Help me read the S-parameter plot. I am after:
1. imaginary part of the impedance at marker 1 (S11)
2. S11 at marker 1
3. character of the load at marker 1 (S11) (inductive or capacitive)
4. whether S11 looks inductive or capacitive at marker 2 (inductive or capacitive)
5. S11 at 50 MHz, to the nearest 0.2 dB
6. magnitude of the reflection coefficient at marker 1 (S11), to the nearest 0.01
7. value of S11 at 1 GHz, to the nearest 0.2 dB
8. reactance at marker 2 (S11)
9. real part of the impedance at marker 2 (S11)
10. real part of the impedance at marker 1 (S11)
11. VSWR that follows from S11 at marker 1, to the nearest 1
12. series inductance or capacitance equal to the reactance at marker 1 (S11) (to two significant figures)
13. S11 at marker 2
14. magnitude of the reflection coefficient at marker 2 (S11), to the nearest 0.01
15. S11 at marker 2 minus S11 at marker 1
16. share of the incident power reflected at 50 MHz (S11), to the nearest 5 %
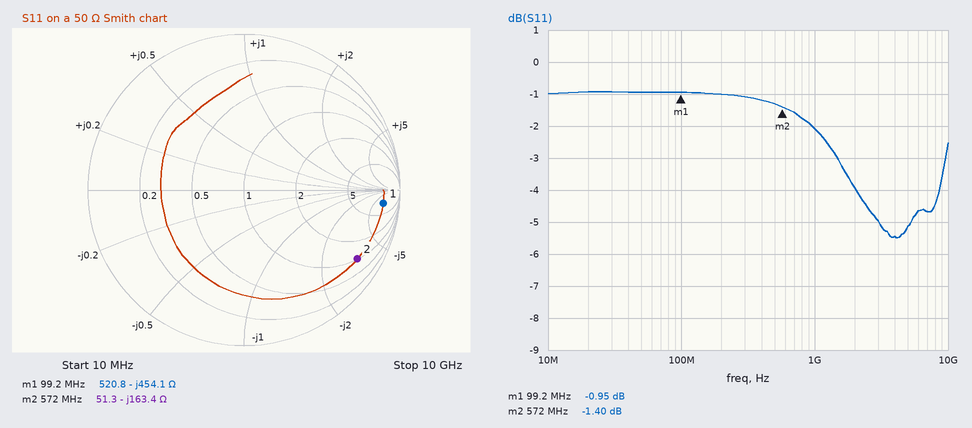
-454.1 Ω
-0.95 dB
capacitive
capacitive
-1.0 dB
0.90
-2.0 dB
-163.4 Ω
51.3 Ω
520.8 Ω
18
3.5 pF
-1.40 dB
0.85
-0.45 dB
80 %
